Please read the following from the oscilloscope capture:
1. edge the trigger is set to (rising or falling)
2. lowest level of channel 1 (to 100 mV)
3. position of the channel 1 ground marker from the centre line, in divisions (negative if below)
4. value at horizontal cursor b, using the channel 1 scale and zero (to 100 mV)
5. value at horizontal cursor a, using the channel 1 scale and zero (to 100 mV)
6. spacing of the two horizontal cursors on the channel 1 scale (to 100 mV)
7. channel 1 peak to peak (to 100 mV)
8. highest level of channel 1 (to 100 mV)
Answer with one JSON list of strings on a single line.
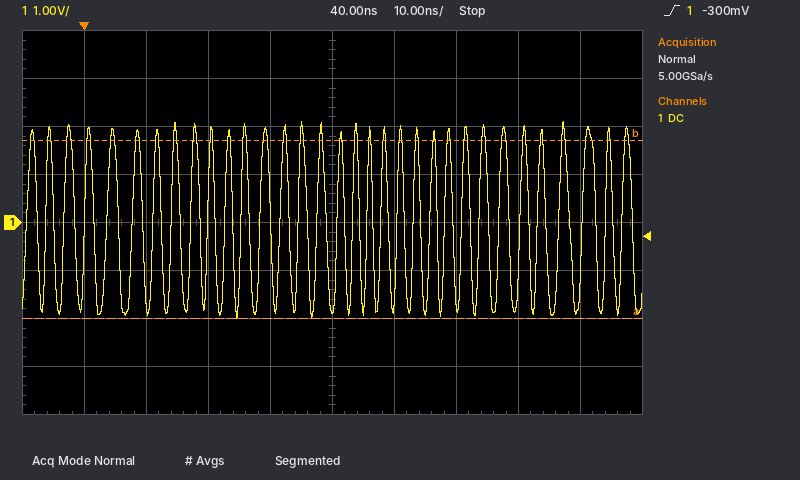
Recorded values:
["rising", "-2.0 V", "0.0 div", "1.7 V", "-2.0 V", "3.7 V", "4.1 V", "2.1 V"]
